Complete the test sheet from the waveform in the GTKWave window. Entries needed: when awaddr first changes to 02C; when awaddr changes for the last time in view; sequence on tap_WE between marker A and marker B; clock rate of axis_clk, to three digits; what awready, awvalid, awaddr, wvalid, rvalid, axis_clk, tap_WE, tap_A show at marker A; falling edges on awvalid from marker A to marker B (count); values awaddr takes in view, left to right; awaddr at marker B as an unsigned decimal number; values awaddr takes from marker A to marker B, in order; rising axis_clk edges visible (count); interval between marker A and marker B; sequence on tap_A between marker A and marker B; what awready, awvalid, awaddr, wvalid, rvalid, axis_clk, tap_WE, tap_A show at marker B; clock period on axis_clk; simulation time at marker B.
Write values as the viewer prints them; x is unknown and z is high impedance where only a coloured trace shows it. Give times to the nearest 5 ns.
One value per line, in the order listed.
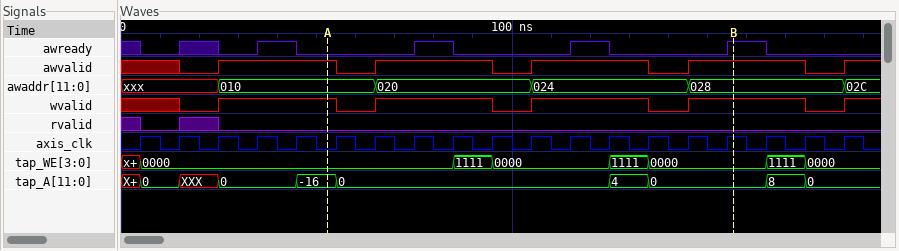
185 ns
185 ns
0000, 1111, 0000, 1111, 0000
100 MHz
awready=0, awvalid=1, awaddr=010, wvalid=1, rvalid=0, axis_clk=0, tap_WE=0000, tap_A=-16
3
xxx, 010, 020, 024, 028, 02C
40
010, 020, 024, 028
19
105 ns
-16, 0, 4, 0
awready=1, awvalid=1, awaddr=028, wvalid=1, rvalid=0, axis_clk=1, tap_WE=0000, tap_A=0
10 ns
155 ns
